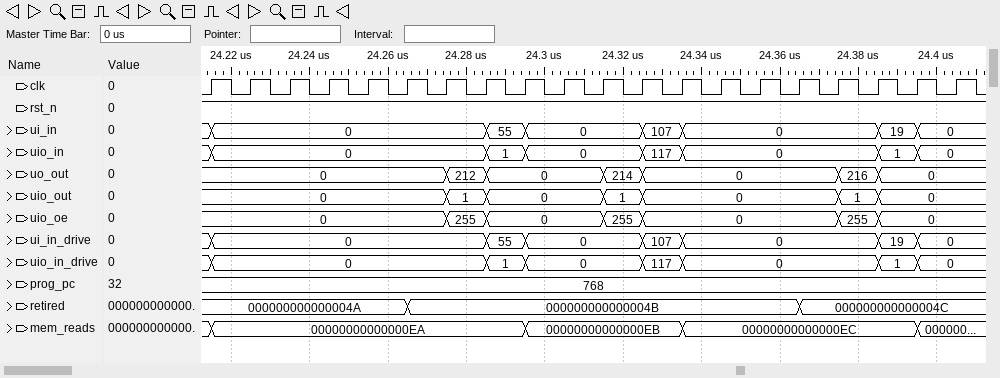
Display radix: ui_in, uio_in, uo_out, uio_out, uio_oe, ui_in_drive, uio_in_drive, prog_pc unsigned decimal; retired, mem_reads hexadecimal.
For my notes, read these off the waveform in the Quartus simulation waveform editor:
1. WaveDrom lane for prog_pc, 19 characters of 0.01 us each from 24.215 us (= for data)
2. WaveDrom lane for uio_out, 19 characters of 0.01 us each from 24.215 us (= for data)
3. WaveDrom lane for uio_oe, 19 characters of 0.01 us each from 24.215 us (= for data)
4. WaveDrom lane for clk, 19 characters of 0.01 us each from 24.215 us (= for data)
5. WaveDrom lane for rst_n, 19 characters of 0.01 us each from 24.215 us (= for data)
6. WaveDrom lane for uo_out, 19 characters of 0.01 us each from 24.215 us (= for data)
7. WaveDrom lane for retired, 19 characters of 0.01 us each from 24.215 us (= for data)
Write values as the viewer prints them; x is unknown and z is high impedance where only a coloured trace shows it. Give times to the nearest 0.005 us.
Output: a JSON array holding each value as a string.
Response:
["{name: 'prog_pc', wave: '=..................', data: '768'}", "{name: 'uio_out', wave: '=.....==..==....==.', data: '0 1 0 1 0 1 0'}", "{name: 'uio_oe', wave: '=.....==..==....==.', data: '0 255 0 255 0 255 0'}", "{name: 'clk', wave: 'p..................'}", "{name: 'rst_n', wave: '1..................'}", "{name: 'uo_out', wave: '=.....==..==....==.', data: '0 212 0 214 0 216 0'}", "{name: 'retired', wave: '=....=.........=...', data: '000000000000004A 000000000000004B 000000000000004C'}"]
